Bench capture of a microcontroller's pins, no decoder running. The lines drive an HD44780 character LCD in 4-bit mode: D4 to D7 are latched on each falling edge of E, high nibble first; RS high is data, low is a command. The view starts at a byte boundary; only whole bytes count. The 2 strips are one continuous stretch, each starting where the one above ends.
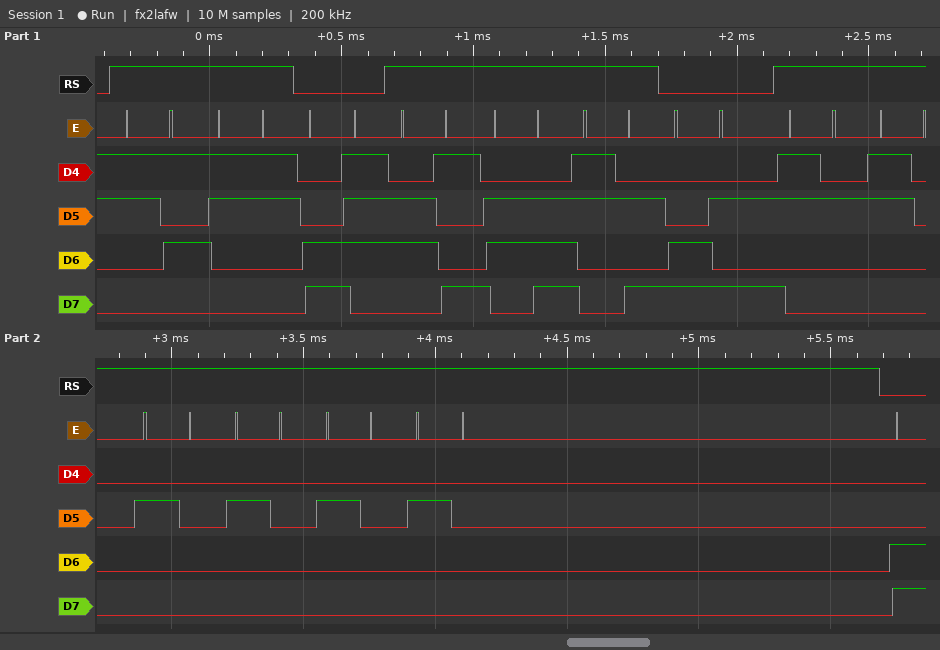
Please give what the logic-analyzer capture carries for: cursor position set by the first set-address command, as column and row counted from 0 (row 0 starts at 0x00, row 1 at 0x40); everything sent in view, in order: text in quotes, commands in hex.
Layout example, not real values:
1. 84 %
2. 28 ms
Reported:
1. column 7, row 1
2. "53" 0xC7 "in:" 0xCA "20    "
